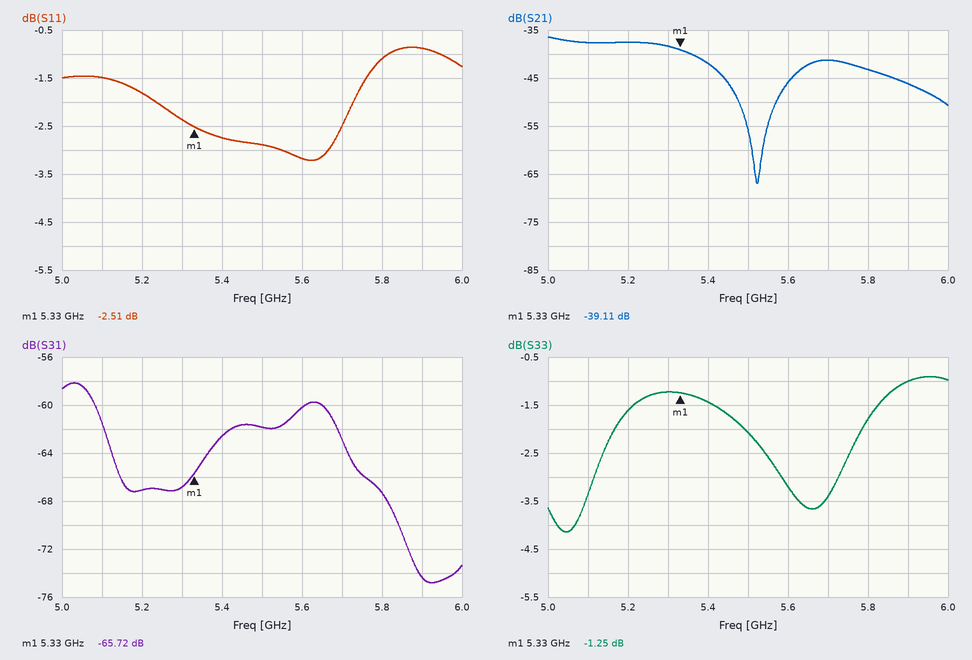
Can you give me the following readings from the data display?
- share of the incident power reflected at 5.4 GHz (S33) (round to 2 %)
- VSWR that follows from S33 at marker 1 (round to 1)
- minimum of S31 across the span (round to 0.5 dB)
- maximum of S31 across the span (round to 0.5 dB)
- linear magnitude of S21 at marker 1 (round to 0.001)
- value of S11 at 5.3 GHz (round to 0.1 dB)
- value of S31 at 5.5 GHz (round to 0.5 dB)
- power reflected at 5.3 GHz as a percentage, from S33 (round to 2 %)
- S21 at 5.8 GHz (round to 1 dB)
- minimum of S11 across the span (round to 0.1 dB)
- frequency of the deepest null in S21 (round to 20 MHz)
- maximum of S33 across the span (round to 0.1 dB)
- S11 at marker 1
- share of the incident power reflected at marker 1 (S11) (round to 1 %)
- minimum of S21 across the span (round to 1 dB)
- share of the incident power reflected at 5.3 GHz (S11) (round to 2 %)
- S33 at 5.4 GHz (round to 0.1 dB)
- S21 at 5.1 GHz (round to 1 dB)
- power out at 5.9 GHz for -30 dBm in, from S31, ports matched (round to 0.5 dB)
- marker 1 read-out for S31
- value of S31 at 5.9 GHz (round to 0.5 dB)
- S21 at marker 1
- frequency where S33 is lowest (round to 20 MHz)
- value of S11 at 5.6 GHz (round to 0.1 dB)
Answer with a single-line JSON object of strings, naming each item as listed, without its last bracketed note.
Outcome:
{"share of the incident power reflected at 5.4 GHz (S33)": "72 %", "VSWR that follows from S33 at marker 1": "14", "minimum of S31 across the span": "-75.0 dB", "maximum of S31 across the span": "-58.0 dB", "linear magnitude of S21 at marker 1": "0.011", "value of S11 at 5.3 GHz": "-2.4 dB", "value of S31 at 5.5 GHz": "-62.0 dB", "power reflected at 5.3 GHz as a percentage, from S33": "76 %", "S21 at 5.8 GHz": "-43 dB", "minimum of S11 across the span": "-3.2 dB", "frequency of the deepest null in S21": "5.52 GHz", "maximum of S33 across the span": "-0.9 dB", "S11 at marker 1": "-2.51 dB", "share of the incident power reflected at marker 1 (S11)": "56 %", "minimum of S21 across the span": "-67 dB", "share of the incident power reflected at 5.3 GHz (S11)": "58 %", "S33 at 5.4 GHz": "-1.4 dB", "S21 at 5.1 GHz": "-38 dB", "power out at 5.9 GHz for -30 dBm in, from S31, ports matched": "-104.5 dBm", "marker 1 read-out for S31": "-65.72 dB", "value of S31 at 5.9 GHz": "-74.5 dB", "S21 at marker 1": "-39.11 dB", "frequency where S33 is lowest": "5.04 GHz", "value of S11 at 5.6 GHz": "-3.2 dB"}
